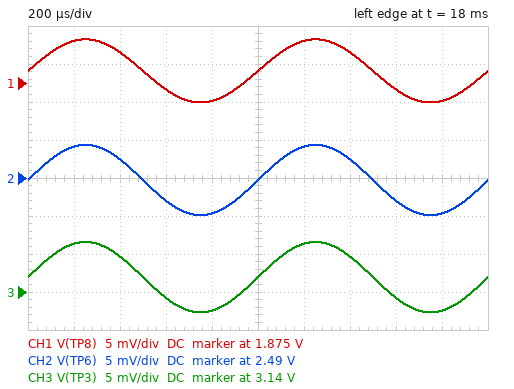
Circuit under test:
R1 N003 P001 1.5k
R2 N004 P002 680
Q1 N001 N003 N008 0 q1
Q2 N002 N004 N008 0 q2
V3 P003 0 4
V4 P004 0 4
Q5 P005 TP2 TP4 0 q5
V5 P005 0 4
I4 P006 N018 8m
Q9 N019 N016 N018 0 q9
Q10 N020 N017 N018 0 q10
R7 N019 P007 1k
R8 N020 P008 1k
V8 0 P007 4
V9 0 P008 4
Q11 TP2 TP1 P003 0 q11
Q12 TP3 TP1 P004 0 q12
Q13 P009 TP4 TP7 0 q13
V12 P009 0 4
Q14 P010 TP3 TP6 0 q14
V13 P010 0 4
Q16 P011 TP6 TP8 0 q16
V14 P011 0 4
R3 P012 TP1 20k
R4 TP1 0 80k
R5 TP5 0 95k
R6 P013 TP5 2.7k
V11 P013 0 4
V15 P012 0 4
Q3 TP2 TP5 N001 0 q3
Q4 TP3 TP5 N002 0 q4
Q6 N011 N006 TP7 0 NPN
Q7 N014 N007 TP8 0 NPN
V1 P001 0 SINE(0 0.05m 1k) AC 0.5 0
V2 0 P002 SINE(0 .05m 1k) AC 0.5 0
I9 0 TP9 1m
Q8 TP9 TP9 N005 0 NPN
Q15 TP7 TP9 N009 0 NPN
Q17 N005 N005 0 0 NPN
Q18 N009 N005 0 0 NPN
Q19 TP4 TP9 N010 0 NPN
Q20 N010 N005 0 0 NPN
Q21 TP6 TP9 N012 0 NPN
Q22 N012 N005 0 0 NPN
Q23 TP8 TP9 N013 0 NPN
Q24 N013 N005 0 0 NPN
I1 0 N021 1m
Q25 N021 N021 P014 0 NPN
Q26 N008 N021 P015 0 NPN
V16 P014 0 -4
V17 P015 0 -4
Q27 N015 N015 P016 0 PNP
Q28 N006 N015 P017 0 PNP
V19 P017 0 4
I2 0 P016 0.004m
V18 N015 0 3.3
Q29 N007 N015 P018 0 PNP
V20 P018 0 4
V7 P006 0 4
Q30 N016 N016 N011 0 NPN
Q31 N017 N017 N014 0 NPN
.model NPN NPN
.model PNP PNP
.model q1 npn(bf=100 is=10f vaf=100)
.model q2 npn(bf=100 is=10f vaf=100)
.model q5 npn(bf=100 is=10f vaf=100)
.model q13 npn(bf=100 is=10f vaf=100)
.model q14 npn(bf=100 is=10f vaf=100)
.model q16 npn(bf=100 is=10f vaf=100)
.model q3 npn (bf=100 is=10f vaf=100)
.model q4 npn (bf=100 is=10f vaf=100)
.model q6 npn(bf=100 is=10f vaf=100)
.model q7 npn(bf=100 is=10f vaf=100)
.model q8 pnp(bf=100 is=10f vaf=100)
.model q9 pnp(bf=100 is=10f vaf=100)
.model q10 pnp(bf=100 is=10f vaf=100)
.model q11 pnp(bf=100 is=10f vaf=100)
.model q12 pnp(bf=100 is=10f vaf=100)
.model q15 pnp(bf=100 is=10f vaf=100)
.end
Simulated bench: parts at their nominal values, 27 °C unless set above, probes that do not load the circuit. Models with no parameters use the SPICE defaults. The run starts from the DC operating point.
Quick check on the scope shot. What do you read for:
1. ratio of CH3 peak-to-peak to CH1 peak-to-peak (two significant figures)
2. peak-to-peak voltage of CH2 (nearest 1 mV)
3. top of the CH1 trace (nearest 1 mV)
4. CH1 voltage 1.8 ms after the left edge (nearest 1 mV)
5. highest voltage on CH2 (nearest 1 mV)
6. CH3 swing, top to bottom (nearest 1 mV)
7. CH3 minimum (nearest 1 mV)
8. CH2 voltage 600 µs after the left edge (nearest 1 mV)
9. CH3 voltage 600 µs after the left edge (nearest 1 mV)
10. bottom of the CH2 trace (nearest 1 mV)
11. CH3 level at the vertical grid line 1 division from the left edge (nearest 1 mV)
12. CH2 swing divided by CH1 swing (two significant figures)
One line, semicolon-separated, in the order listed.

1.1; 9 mV; 1.881 V; 1.873 V; 2.494 V; 9 mV; 3.137 V; 2.487 V; 3.139 V; 2.485 V; 3.146 V; 1.1
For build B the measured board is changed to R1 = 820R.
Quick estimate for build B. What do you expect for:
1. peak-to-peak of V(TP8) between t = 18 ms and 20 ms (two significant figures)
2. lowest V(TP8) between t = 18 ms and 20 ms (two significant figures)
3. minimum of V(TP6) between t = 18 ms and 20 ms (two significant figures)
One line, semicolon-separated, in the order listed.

18 mV; 2.0 V; 2.7 V
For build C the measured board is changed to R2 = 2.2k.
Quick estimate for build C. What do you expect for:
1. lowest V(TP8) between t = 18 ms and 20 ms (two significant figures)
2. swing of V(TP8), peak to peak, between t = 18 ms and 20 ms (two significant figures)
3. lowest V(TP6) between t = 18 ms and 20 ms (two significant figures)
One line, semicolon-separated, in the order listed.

2.5 V; 1.0 mV; 3.2 V
